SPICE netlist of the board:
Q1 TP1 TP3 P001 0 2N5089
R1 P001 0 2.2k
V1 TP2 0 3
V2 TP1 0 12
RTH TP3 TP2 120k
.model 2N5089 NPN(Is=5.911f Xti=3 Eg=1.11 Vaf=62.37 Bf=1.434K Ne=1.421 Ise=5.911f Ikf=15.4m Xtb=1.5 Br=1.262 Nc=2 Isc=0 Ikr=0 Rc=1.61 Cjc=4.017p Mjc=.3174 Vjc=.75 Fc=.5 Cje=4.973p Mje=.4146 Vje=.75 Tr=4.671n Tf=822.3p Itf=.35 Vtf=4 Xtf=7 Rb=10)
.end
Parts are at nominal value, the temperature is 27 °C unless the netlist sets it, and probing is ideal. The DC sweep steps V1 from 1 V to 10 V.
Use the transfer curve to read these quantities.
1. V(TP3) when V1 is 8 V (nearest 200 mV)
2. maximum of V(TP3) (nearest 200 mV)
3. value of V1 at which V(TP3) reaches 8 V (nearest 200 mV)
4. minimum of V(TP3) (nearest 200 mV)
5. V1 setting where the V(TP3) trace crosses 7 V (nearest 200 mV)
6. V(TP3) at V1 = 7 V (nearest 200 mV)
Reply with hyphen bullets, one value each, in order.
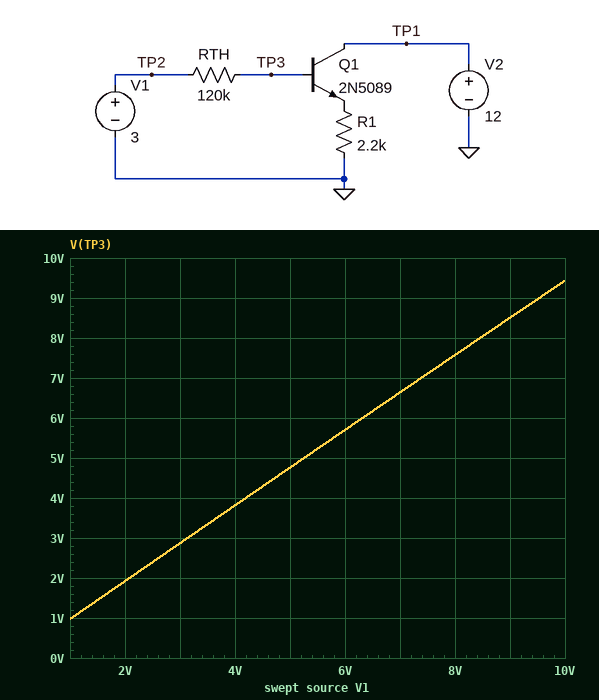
- 7.6 V
- 9.4 V
- 8.4 V
- 1.0 V
- 7.4 V
- 6.6 V
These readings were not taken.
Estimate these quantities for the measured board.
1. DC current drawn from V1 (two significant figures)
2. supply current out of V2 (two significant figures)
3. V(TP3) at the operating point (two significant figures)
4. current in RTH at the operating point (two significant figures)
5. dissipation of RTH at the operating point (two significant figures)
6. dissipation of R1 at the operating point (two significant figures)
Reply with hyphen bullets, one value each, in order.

- 1.1 µA
- 1.0 mA
- 2.9 V
- 1.1 µA
- 140 nW
- 2.2 mW
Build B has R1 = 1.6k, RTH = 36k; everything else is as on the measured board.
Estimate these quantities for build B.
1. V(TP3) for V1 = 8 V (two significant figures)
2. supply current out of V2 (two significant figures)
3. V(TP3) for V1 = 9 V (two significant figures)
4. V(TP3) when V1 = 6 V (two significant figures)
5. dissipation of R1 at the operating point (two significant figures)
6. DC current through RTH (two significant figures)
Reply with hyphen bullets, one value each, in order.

- 7.8 V
- 1.4 mA
- 8.8 V
- 5.9 V
- 3.2 mW
- 1.5 µA
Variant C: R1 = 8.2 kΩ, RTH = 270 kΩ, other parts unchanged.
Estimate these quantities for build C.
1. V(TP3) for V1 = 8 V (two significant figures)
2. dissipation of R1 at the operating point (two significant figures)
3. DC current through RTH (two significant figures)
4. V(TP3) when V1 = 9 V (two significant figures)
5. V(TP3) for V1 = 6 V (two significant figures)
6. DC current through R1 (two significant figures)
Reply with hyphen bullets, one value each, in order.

- 7.7 V
- 630 µW
- 350 nA
- 8.7 V
- 5.8 V
- 280 µA
